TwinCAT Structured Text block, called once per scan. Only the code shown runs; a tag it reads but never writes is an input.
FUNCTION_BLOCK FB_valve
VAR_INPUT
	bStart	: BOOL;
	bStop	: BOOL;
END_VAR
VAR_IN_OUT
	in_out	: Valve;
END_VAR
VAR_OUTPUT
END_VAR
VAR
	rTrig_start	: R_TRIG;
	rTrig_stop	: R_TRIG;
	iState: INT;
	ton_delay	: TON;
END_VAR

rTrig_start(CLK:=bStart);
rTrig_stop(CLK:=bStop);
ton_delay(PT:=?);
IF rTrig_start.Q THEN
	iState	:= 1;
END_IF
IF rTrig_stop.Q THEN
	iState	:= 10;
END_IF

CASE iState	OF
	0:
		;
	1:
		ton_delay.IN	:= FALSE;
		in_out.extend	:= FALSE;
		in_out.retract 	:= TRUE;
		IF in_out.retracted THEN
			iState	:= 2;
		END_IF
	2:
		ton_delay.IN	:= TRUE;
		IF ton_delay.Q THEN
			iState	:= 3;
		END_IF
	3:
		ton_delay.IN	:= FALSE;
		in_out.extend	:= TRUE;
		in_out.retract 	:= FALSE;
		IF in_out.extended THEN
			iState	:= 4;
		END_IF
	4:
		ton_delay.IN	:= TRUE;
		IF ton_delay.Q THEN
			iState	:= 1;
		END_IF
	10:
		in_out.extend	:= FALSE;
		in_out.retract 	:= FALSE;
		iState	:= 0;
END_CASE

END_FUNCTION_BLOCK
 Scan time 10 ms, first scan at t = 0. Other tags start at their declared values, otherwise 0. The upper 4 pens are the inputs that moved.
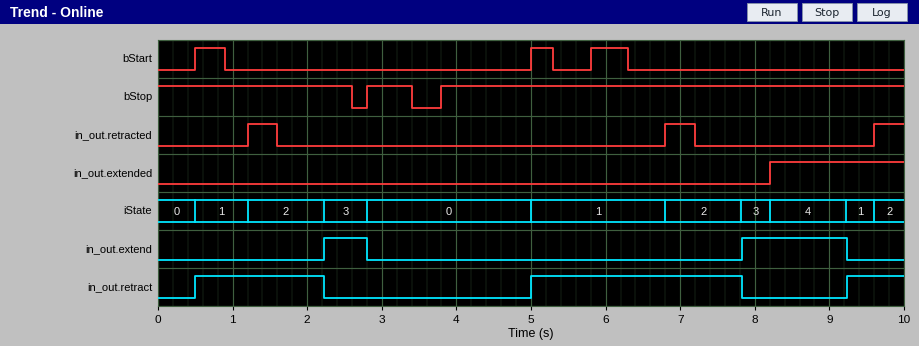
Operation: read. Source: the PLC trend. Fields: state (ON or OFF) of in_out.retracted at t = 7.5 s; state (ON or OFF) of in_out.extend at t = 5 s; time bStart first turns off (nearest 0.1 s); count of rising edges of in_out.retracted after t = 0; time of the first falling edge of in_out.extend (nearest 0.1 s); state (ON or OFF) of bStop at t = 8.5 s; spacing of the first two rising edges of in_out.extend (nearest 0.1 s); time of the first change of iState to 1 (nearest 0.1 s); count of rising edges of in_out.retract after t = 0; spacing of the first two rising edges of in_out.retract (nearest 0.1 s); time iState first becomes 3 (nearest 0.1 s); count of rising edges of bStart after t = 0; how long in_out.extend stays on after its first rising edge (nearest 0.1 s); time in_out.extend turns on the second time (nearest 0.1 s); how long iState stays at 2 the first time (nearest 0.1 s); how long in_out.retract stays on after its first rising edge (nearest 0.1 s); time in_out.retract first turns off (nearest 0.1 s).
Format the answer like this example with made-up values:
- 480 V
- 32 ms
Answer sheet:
- OFF
- OFF
- 0.9 s
- 3
- 2.8 s
- ON
- 5.6 s
- 0.5 s
- 3
- 4.5 s
- 2.2 s
- 3
- 0.6 s
- 7.8 s
- 1.0 s
- 1.7 s
- 2.2 s
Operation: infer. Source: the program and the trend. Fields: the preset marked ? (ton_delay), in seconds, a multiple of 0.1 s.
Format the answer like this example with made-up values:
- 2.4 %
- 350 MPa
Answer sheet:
- 1.0 s
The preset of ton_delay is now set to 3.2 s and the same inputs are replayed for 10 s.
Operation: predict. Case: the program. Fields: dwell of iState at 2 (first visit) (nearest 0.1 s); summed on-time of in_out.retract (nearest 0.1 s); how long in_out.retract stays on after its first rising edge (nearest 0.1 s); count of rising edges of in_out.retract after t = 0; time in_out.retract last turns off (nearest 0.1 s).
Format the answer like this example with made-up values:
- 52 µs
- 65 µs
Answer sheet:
- 1.6 s
- 7.3 s
- 2.3 s
- 2
- 2.8 s
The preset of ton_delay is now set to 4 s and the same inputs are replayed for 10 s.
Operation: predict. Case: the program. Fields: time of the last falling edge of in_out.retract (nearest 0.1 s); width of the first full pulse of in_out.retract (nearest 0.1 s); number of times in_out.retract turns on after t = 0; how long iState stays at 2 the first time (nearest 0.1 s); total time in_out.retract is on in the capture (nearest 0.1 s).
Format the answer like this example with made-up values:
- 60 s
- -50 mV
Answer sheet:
- 2.8 s
- 2.3 s
- 2
- 1.6 s
- 7.3 s
